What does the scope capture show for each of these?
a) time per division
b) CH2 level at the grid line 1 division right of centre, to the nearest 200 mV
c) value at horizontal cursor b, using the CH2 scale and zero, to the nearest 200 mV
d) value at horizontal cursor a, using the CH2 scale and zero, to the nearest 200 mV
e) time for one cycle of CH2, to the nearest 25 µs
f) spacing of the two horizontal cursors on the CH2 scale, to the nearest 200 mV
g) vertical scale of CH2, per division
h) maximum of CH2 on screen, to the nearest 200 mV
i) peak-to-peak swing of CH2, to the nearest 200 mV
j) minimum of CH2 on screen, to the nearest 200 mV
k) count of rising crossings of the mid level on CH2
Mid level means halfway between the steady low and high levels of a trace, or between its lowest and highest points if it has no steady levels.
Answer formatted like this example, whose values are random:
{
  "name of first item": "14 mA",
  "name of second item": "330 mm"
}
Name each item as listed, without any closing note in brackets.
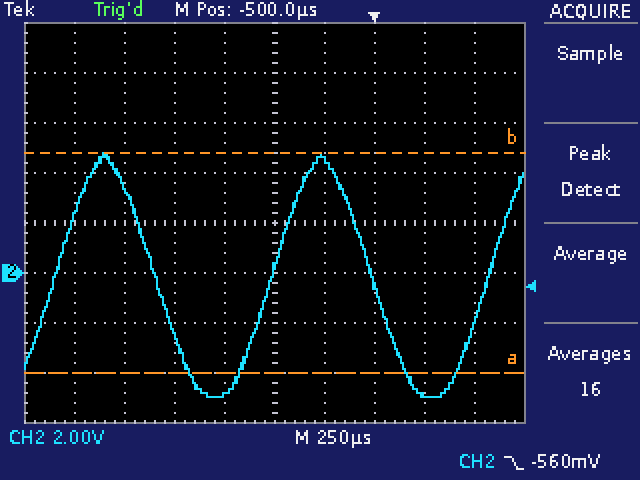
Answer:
{
  "time per division": "250 µs",
  "CH2 level at the grid line 1 division right of centre, to the nearest 200 mV": "4.6 V",
  "value at horizontal cursor b, using the CH2 scale and zero, to the nearest 200 mV": "4.8 V",
  "value at horizontal cursor a, using the CH2 scale and zero, to the nearest 200 mV": "-4.0 V",
  "time for one cycle of CH2, to the nearest 25 µs": "1.075 ms",
  "spacing of the two horizontal cursors on the CH2 scale, to the nearest 200 mV": "8.8 V",
  "vertical scale of CH2, per division": "2 V",
  "maximum of CH2 on screen, to the nearest 200 mV": "4.8 V",
  "peak-to-peak swing of CH2, to the nearest 200 mV": "9.8 V",
  "minimum of CH2 on screen, to the nearest 200 mV": "-5.0 V",
  "count of rising crossings of the mid level on CH2": "3"
}
